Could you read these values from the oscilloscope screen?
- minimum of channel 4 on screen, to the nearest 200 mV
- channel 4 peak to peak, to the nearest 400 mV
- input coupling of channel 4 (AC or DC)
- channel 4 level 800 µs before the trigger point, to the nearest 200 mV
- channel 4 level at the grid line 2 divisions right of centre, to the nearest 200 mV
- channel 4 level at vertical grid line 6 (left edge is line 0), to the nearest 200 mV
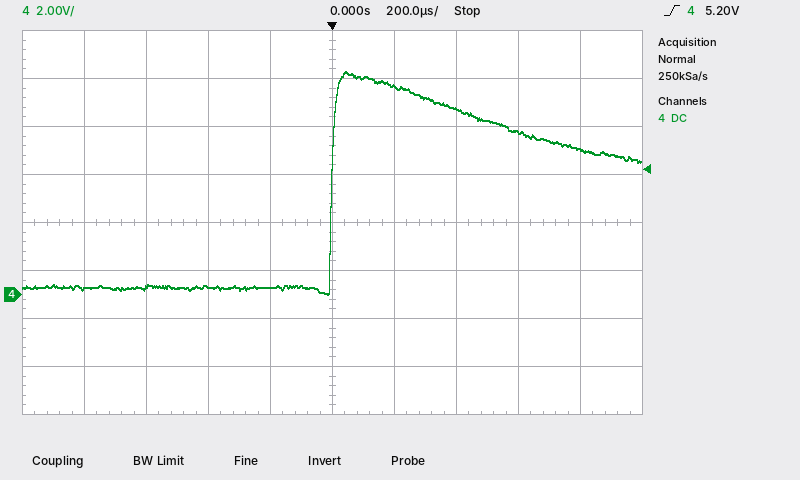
0.0 V
9.2 V
DC
200 mV
7.8 V
8.6 V
